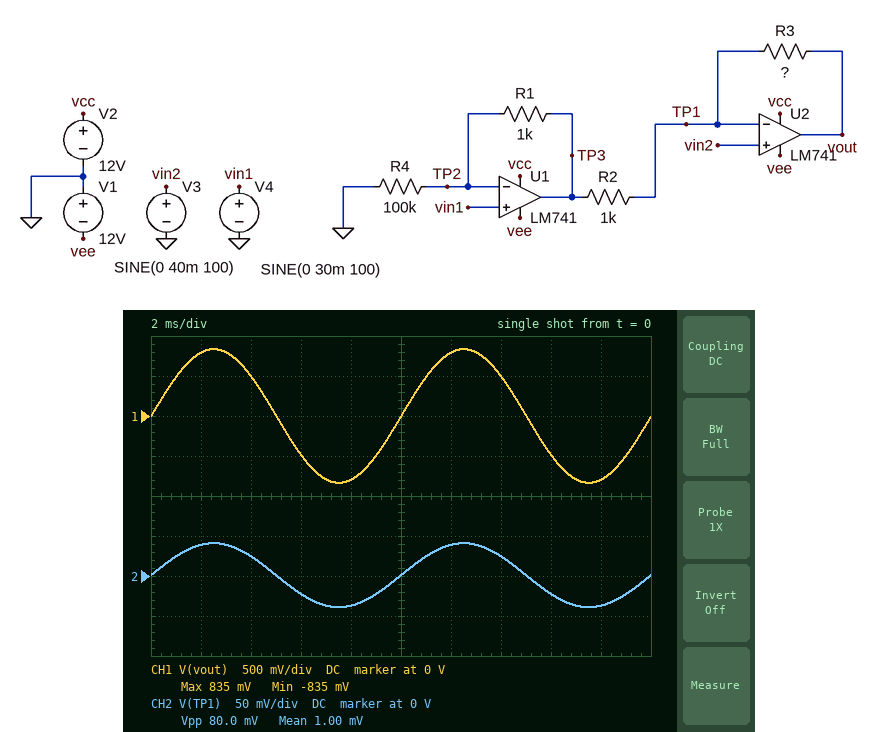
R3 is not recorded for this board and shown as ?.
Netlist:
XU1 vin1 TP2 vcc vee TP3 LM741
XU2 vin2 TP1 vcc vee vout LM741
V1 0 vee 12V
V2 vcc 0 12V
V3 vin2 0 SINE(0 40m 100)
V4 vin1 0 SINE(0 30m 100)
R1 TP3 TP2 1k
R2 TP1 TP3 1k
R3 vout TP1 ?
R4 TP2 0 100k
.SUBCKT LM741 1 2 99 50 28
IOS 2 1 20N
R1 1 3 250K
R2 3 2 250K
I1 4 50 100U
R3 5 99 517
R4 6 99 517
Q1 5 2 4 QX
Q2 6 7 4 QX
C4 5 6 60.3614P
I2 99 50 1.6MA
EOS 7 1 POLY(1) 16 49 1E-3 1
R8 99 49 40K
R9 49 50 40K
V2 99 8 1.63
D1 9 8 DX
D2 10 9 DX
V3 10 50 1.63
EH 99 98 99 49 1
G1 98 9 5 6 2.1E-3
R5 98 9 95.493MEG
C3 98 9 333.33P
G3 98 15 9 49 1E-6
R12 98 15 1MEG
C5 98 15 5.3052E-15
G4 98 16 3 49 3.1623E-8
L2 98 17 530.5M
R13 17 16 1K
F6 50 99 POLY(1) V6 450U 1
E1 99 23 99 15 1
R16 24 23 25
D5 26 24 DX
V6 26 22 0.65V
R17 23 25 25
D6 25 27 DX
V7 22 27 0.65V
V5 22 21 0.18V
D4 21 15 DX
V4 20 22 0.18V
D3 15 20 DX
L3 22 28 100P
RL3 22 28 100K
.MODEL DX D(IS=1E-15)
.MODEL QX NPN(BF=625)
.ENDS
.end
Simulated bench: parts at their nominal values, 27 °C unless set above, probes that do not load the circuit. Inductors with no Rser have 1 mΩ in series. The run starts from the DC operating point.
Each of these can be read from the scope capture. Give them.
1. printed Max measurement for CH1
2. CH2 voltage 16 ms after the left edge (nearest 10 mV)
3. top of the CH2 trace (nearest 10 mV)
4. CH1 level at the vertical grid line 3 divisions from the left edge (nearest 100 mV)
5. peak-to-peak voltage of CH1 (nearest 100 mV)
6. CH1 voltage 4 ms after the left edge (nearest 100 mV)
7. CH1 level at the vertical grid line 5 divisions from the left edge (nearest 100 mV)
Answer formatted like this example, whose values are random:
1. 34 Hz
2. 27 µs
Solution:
1. 835 mV
2. -20 mV
3. 40 mV
4. -500 mV
5. 1.7 V
6. 500 mV
7. 0 V
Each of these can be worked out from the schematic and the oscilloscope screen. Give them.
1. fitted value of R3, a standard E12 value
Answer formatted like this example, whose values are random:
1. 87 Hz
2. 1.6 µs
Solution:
1. 82 kΩ
